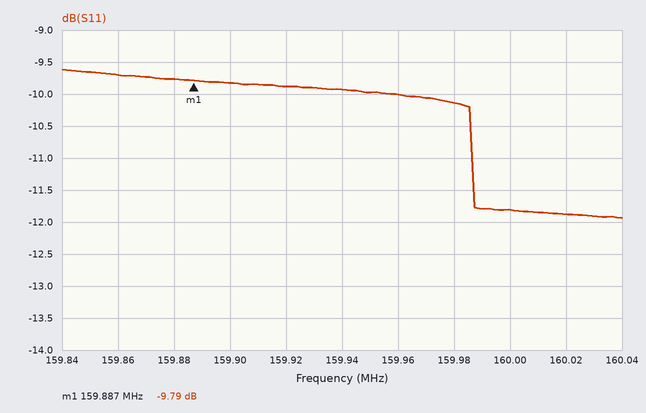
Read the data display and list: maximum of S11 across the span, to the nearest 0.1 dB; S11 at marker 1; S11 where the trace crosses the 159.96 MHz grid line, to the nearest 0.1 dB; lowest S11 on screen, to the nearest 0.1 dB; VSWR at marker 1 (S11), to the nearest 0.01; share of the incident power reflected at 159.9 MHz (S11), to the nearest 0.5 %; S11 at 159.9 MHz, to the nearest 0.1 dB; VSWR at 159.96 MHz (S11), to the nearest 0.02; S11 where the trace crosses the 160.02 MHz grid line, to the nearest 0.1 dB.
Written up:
-9.6 dB
-9.79 dB
-10.0 dB
-11.9 dB
1.96
10.5 %
-9.8 dB
1.92
-11.9 dB
